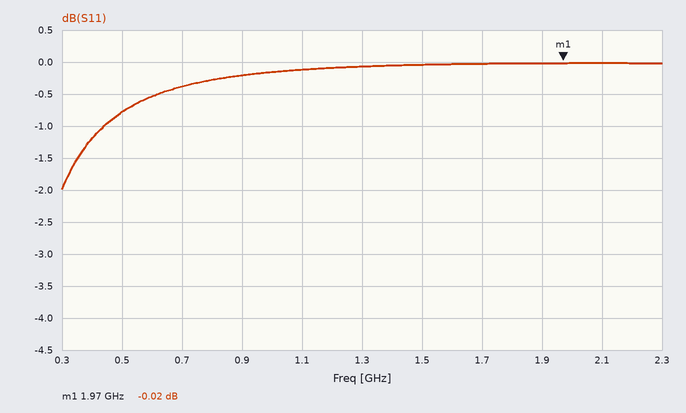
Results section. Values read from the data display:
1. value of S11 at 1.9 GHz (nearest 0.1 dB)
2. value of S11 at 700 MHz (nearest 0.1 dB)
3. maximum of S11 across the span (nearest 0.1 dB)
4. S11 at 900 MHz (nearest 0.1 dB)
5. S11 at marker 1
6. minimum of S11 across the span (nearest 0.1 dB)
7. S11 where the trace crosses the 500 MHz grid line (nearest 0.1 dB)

0.0 dB
-0.4 dB
0.0 dB
-0.2 dB
-0.02 dB
-2.0 dB
-0.8 dB
